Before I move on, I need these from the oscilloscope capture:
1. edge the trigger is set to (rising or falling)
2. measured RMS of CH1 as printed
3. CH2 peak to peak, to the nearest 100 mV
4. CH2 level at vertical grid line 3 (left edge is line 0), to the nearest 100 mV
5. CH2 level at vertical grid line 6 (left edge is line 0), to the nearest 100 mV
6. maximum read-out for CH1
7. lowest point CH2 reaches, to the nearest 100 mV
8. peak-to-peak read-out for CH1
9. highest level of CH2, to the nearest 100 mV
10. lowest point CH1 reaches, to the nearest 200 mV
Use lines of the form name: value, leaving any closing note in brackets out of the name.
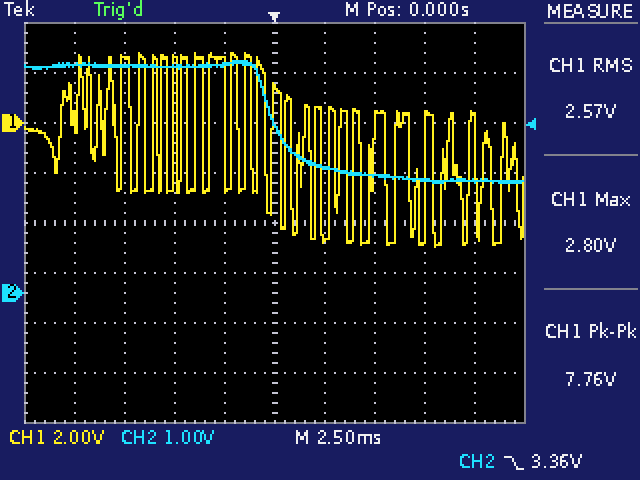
edge the trigger is set to: falling
measured RMS of CH1 as printed: 2.57 V
CH2 peak to peak, to the nearest 100 mV: 2.4 V
CH2 level at vertical grid line 3 (left edge is line 0), to the nearest 100 mV: 4.5 V
CH2 level at vertical grid line 6 (left edge is line 0), to the nearest 100 mV: 2.5 V
maximum read-out for CH1: 2.80 V
lowest point CH2 reaches, to the nearest 100 mV: 2.2 V
peak-to-peak read-out for CH1: 7.76 V
highest level of CH2, to the nearest 100 mV: 4.6 V
lowest point CH1 reaches, to the nearest 200 mV: -5.0 V
